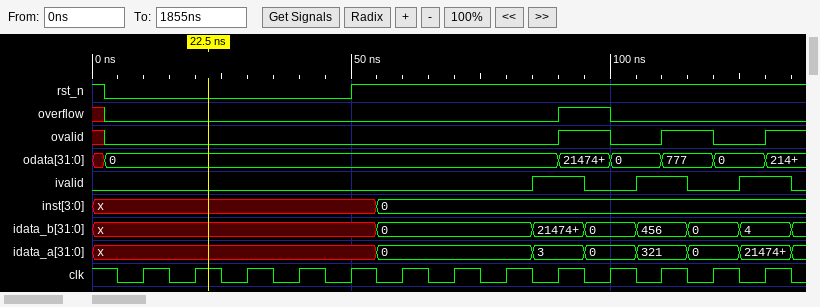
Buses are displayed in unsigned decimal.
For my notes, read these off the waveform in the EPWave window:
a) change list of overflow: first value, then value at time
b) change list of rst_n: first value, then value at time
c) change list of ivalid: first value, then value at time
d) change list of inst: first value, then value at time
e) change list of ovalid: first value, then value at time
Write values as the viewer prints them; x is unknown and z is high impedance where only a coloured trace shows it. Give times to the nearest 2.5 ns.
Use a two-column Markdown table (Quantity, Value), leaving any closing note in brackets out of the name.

| Quantity | Value |
|---|---|
| change list of overflow: first value, then value at time | x, 0 at 2.5 ns, 1 at 90 ns, 0 at 100 ns |
| change list of rst_n: first value, then value at time | 1, 0 at 2.5 ns, 1 at 50 ns |
| change list of ivalid: first value, then value at time | 0, 1 at 85 ns, 0 at 95 ns, 1 at 105 ns, 0 at 115 ns, 1 at 125 ns, 0 at 135 ns |
| change list of inst: first value, then value at time | x, 0 at 55 ns |
| change list of ovalid: first value, then value at time | x, 0 at 2.5 ns, 1 at 90 ns, 0 at 100 ns, 1 at 110 ns, 0 at 120 ns, 1 at 130 ns |
